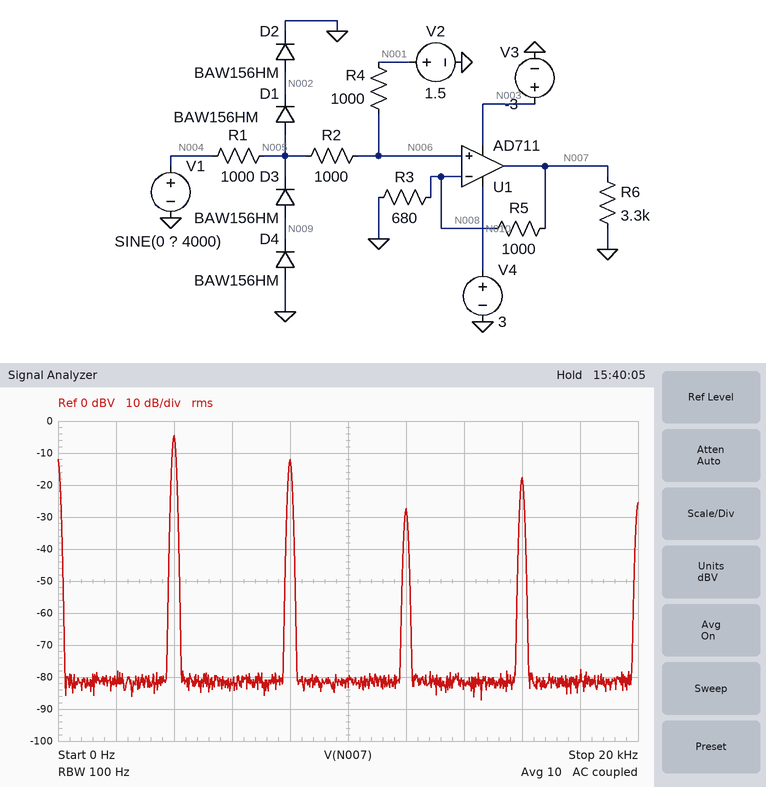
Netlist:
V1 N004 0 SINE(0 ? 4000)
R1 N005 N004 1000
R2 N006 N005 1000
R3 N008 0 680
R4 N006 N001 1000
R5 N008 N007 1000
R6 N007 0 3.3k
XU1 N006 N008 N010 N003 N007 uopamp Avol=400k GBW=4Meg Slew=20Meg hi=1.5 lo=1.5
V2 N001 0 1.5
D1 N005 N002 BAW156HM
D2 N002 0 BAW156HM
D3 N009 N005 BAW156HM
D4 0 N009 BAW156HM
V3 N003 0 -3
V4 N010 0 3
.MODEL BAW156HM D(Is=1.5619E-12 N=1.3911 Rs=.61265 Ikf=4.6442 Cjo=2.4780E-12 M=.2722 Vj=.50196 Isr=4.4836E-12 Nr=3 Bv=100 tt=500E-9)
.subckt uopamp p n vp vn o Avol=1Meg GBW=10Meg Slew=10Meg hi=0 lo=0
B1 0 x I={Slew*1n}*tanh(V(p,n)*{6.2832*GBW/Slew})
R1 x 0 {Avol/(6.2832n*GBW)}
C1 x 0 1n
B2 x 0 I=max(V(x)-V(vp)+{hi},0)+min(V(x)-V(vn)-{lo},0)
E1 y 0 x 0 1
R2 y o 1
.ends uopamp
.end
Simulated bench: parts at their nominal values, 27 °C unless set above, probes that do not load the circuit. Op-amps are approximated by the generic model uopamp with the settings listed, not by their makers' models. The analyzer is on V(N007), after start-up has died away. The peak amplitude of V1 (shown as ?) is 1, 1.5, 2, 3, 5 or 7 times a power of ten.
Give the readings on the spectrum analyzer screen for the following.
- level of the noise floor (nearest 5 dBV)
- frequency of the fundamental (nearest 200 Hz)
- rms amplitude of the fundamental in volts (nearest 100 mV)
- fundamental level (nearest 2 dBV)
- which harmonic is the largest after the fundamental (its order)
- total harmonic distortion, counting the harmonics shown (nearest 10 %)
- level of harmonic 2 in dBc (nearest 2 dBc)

-80 dBV
4.0 kHz
600 mV
-4 dBV
2
50 %
-8 dBc
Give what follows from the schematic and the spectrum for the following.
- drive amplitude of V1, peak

5 V
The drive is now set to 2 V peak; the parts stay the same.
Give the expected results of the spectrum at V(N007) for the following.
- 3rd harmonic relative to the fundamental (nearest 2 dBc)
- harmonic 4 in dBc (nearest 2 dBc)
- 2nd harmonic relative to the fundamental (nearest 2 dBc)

-8 dBc
-16 dBc
-2 dBc
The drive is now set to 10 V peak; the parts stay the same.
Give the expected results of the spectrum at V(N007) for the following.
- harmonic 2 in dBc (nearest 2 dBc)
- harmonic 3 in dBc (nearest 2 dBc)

-12 dBc
-12 dBc
